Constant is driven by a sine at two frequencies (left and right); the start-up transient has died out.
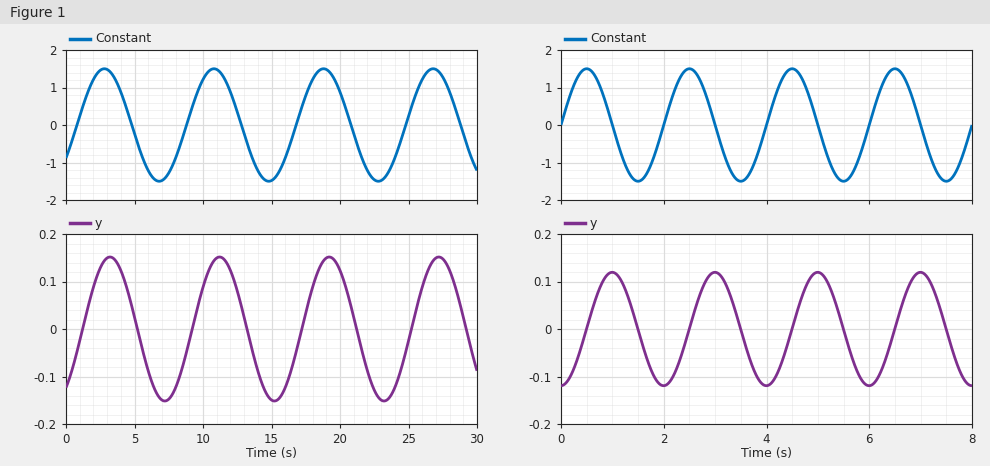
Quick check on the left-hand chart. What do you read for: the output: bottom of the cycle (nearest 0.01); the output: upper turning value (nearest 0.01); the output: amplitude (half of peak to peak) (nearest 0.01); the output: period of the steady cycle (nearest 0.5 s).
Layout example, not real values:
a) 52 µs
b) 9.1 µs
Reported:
a) -0.15
b) 0.15
c) 0.15
d) 8.0 s
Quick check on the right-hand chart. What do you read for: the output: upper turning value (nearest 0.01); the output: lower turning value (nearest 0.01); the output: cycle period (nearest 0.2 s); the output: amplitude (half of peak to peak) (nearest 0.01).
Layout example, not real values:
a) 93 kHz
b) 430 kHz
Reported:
a) 0.12
b) -0.12
c) 2.0 s
d) 0.12
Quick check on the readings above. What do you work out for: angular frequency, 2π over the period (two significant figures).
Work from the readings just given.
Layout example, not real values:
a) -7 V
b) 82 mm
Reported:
a) 3.1 rad/s
